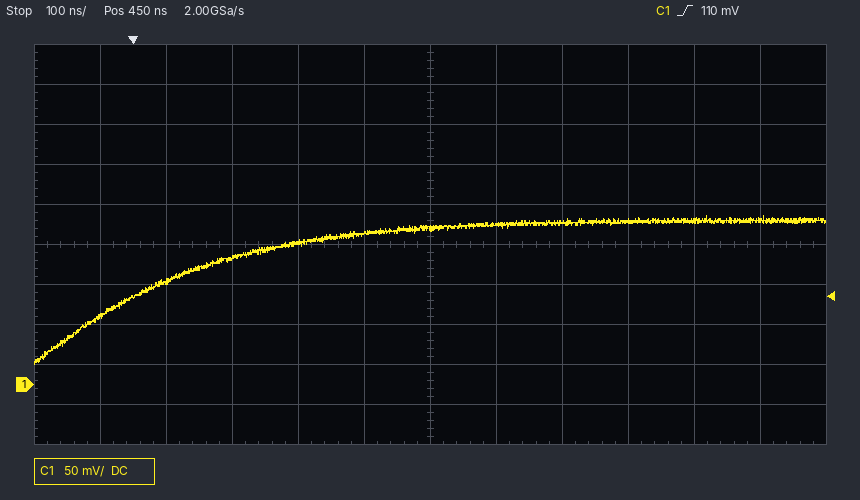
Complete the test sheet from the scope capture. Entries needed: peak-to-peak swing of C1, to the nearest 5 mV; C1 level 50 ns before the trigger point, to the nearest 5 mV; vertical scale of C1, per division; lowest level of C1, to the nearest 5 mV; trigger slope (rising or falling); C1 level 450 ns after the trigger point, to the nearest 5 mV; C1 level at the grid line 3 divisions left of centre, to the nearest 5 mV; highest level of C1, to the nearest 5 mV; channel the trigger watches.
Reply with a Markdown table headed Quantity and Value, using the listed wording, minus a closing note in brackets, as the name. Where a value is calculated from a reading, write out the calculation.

| Quantity | Value |
|---|---|
| peak-to-peak swing of C1, to the nearest 5 mV | 210 mV − (25 mV) = 185 mV |
| C1 level 50 ns before the trigger point, to the nearest 5 mV | 85 mV |
| vertical scale of C1, per division | 50 mV |
| lowest level of C1, to the nearest 5 mV | 25 mV |
| trigger slope | rising |
| C1 level 450 ns after the trigger point, to the nearest 5 mV | 195 mV |
| C1 level at the grid line 3 divisions left of centre, to the nearest 5 mV | 160 mV |
| highest level of C1, to the nearest 5 mV | 210 mV |
| channel the trigger watches | C1 |
